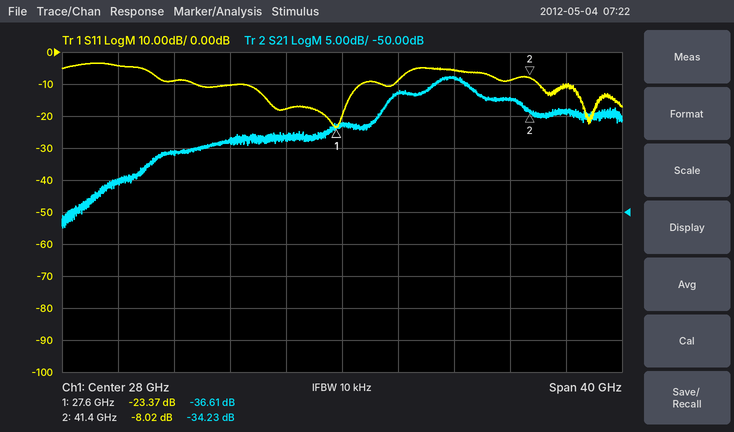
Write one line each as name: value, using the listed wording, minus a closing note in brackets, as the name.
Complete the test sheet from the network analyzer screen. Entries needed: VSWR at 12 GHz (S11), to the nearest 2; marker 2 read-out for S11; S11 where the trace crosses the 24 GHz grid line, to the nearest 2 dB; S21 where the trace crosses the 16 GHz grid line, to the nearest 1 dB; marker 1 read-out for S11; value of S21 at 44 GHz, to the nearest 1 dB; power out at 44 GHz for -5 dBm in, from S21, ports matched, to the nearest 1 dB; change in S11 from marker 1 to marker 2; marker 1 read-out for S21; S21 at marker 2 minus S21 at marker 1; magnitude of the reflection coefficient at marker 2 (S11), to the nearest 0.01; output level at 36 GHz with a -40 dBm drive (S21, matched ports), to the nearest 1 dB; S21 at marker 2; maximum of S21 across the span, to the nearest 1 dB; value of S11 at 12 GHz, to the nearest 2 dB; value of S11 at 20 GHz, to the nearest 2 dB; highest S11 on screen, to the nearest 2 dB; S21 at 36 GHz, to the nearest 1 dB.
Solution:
VSWR at 12 GHz (S11), to the nearest 2: 4
marker 2 read-out for S11: -8.02 dB
S11 where the trace crosses the 24 GHz grid line, to the nearest 2 dB: -18 dB
S21 where the trace crosses the 16 GHz grid line, to the nearest 1 dB: -41 dB
marker 1 read-out for S11: -23.37 dB
value of S21 at 44 GHz, to the nearest 1 dB: -34 dB
power out at 44 GHz for -5 dBm in, from S21, ports matched, to the nearest 1 dB: -39 dBm
change in S11 from marker 1 to marker 2: 15.35 dB
marker 1 read-out for S21: -36.61 dB
S21 at marker 2 minus S21 at marker 1: 2.38 dB
magnitude of the reflection coefficient at marker 2 (S11), to the nearest 0.01: 0.40
output level at 36 GHz with a -40 dBm drive (S21, matched ports), to the nearest 1 dB: -69 dBm
S21 at marker 2: -34.23 dB
maximum of S21 across the span, to the nearest 1 dB: -29 dB
value of S11 at 12 GHz, to the nearest 2 dB: -4 dB
value of S11 at 20 GHz, to the nearest 2 dB: -10 dB
highest S11 on screen, to the nearest 2 dB: -4 dB
S21 at 36 GHz, to the nearest 1 dB: -29 dB
